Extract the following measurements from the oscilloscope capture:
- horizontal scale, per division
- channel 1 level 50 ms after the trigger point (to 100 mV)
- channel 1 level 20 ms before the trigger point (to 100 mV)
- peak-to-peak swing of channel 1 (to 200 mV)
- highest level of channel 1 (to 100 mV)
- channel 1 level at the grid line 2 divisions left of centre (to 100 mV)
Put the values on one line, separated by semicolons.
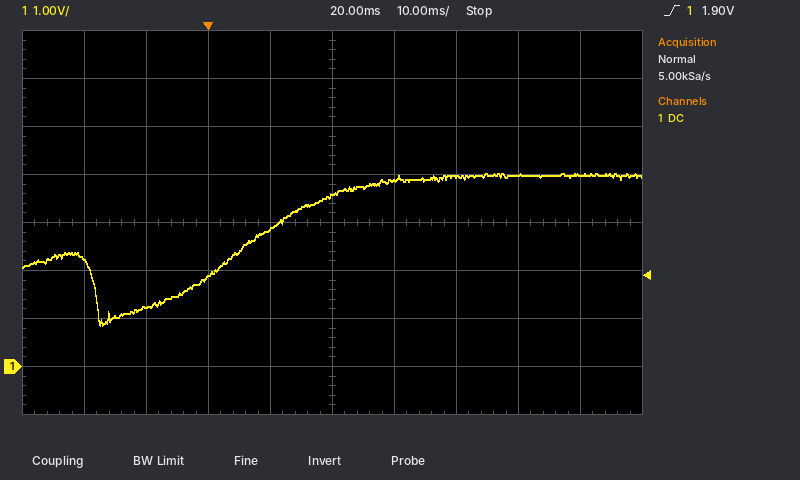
10 ms; 4.0 V; 2.2 V; 3.2 V; 4.0 V; 1.9 V
